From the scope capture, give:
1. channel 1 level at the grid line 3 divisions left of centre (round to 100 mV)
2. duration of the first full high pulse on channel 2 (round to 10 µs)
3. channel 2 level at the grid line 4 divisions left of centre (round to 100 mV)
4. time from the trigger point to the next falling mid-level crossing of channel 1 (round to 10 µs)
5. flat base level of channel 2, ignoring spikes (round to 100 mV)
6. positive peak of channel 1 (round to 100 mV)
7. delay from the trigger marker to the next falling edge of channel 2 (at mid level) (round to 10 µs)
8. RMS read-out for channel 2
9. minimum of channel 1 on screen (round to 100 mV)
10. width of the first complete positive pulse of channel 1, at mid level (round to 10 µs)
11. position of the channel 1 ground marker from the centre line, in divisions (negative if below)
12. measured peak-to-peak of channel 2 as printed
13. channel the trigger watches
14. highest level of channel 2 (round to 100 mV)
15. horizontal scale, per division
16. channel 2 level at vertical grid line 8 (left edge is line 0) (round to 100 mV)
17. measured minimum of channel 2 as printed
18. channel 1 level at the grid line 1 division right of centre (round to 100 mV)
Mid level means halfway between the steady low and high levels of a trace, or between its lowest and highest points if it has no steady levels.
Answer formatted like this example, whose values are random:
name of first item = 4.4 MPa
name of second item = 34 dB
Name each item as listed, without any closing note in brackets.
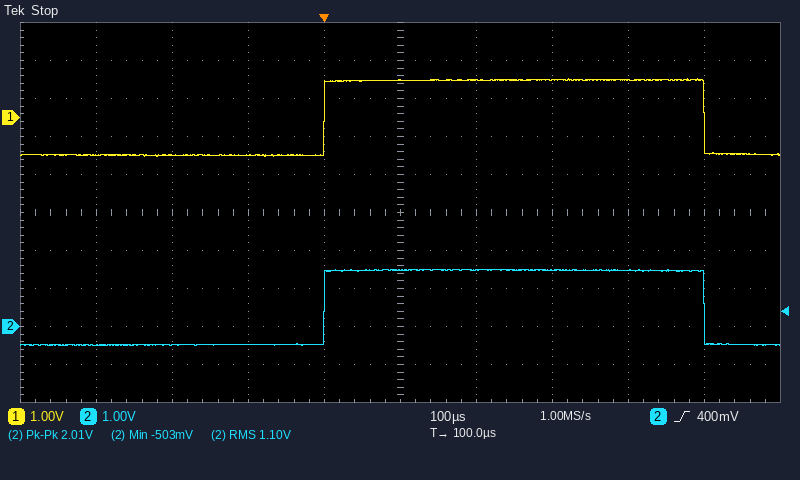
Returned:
channel 1 level at the grid line 3 divisions left of centre = -1.0 V
duration of the first full high pulse on channel 2 = 500 µs
channel 2 level at the grid line 4 divisions left of centre = -500 mV
time from the trigger point to the next falling mid-level crossing of channel 1 = 500 µs
flat base level of channel 2, ignoring spikes = -500 mV
positive peak of channel 1 = 1.0 V
delay from the trigger marker to the next falling edge of channel 2 (at mid level) = 500 µs
RMS read-out for channel 2 = 1.10 V
minimum of channel 1 on screen = -1.0 V
width of the first complete positive pulse of channel 1, at mid level = 500 µs
position of the channel 1 ground marker from the centre line, in divisions = +2.5 div
measured peak-to-peak of channel 2 as printed = 2.01 V
channel the trigger watches = channel 2
highest level of channel 2 = 1.5 V
horizontal scale, per division = 100 µs
channel 2 level at vertical grid line 8 (left edge is line 0) = 1.5 V
measured minimum of channel 2 as printed = -503 mV
channel 1 level at the grid line 1 division right of centre = 1.0 V
